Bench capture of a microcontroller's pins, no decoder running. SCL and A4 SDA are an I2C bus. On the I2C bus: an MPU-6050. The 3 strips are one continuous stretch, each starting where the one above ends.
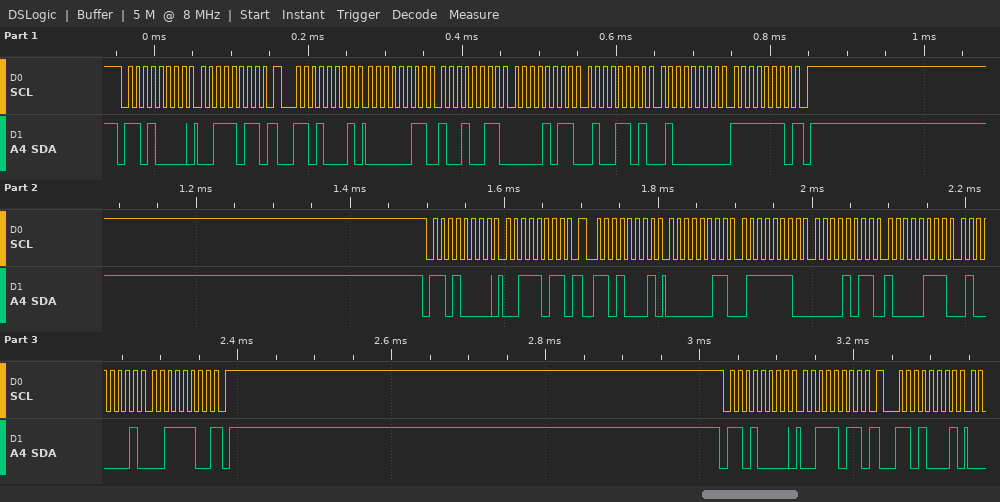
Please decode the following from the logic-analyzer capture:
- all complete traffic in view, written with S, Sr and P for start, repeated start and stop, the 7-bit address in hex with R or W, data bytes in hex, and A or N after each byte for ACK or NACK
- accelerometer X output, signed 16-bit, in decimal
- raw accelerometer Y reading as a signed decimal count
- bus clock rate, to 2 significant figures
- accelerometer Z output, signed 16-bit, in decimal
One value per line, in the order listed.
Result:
S 68W A 3B A Sr 68R A 03 A 93 A 0B A 4D A 40 A FE N P S 68W A 3B A Sr 68R A 03 A 7E A 0B A 87 A 41 A 3C N P S 68W A 3B A Sr 68R A
915
2893
100 kHz
16638
